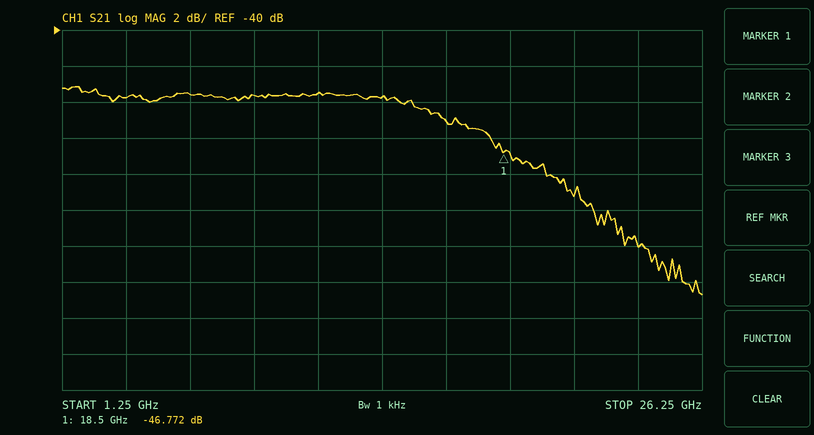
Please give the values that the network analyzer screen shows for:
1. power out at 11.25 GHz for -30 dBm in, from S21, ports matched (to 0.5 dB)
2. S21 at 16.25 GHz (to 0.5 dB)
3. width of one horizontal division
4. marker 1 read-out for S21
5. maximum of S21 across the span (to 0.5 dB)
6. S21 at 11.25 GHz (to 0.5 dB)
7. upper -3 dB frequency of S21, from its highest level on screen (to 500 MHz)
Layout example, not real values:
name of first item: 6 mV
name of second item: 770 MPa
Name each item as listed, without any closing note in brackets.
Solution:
power out at 11.25 GHz for -30 dBm in, from S21, ports matched: -73.5 dBm
S21 at 16.25 GHz: -45.0 dB
width of one horizontal division: 2.5 GHz
marker 1 read-out for S21: -46.772 dB
maximum of S21 across the span: -43.0 dB
S21 at 11.25 GHz: -43.5 dB
upper -3 dB frequency of S21, from its highest level on screen: 18.0 GHz
